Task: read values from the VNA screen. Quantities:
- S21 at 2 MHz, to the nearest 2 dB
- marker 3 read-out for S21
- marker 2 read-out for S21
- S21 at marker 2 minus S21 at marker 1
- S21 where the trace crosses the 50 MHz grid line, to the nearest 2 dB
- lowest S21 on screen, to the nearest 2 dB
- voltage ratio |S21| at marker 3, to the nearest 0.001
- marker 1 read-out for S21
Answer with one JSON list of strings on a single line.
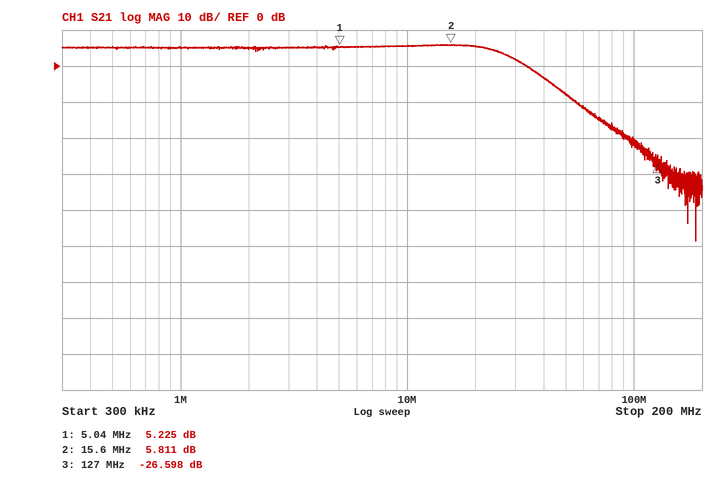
["4 dB", "-26.598 dB", "5.811 dB", "0.586 dB", "-8 dB", "-48 dB", "0.047", "5.225 dB"]
